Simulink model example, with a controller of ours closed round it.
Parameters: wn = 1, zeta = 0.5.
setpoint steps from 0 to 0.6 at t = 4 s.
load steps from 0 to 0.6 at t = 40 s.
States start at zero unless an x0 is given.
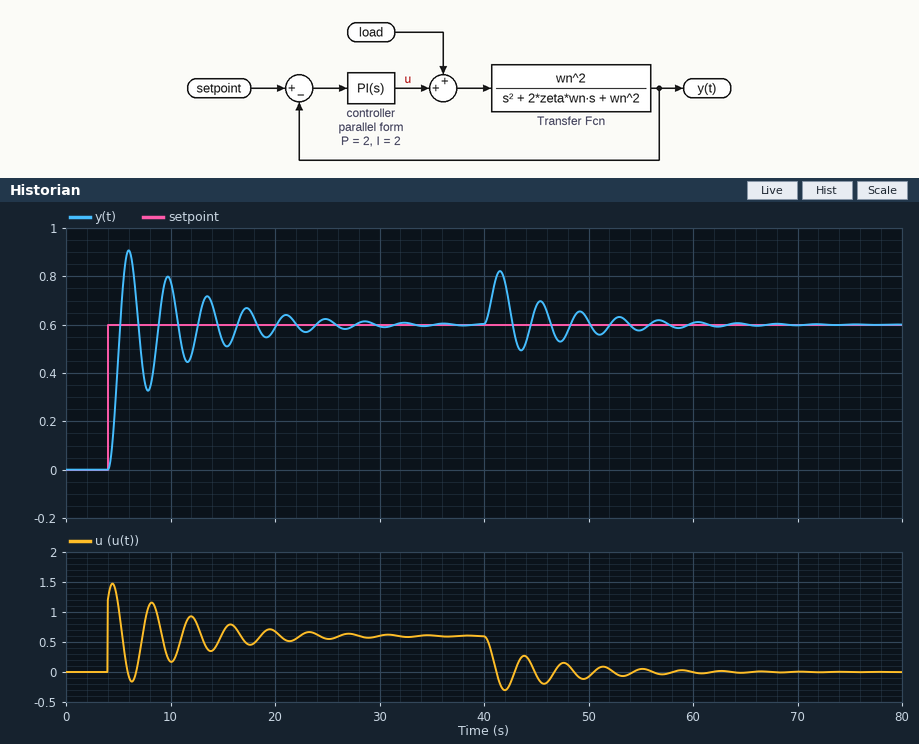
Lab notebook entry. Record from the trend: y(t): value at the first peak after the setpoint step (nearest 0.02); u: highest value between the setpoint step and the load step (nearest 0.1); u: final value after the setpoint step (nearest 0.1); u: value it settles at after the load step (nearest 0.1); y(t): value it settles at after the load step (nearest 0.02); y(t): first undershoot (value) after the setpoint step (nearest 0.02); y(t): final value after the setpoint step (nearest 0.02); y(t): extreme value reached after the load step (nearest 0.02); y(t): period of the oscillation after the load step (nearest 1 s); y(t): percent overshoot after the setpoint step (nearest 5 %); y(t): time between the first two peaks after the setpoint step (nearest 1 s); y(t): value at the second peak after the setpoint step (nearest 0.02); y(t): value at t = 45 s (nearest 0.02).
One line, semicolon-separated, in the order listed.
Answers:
0.90; 1.5; 0.6; 0.0; 0.60; 0.32; 0.60; 0.82; 4 s; 50 %; 4 s; 0.80; 0.68
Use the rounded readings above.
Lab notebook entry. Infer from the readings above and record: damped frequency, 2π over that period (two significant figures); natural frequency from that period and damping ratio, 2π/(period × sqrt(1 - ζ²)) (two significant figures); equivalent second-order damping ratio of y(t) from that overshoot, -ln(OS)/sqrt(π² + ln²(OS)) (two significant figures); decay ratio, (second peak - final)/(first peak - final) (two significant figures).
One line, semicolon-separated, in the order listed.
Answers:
1.6 rad/s; 1.6 rad/s; 0.22; 0.67
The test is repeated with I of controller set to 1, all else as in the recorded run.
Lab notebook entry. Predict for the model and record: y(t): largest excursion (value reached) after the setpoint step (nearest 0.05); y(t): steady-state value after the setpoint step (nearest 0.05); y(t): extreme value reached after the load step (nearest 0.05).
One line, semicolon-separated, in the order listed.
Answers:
0.75; 0.60; 0.85
